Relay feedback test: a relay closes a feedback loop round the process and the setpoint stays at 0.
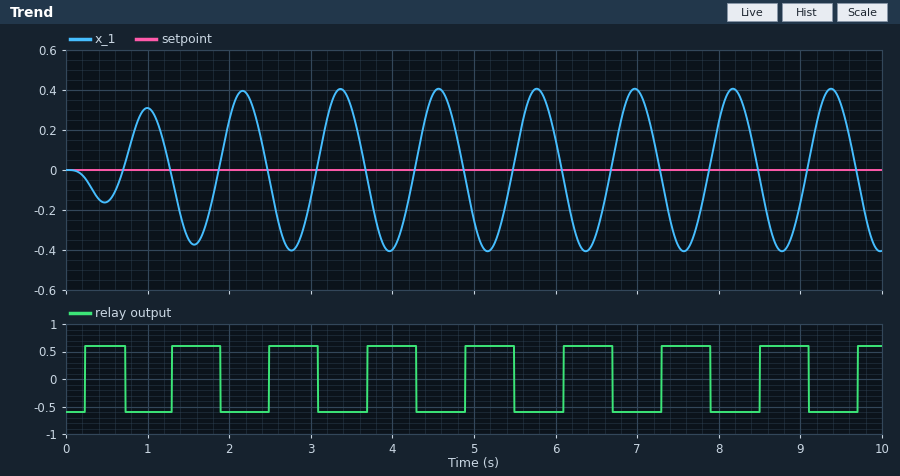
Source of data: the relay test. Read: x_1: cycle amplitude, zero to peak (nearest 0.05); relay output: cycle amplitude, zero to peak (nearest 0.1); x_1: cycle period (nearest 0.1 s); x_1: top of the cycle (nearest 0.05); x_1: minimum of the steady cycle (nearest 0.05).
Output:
0.40
0.6
1.2 s
0.40
-0.40
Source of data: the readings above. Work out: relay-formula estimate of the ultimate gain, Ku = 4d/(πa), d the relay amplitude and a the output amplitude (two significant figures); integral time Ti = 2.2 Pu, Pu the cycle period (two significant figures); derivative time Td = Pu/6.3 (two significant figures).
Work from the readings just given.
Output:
1.9
2.6 s
0.19 s
